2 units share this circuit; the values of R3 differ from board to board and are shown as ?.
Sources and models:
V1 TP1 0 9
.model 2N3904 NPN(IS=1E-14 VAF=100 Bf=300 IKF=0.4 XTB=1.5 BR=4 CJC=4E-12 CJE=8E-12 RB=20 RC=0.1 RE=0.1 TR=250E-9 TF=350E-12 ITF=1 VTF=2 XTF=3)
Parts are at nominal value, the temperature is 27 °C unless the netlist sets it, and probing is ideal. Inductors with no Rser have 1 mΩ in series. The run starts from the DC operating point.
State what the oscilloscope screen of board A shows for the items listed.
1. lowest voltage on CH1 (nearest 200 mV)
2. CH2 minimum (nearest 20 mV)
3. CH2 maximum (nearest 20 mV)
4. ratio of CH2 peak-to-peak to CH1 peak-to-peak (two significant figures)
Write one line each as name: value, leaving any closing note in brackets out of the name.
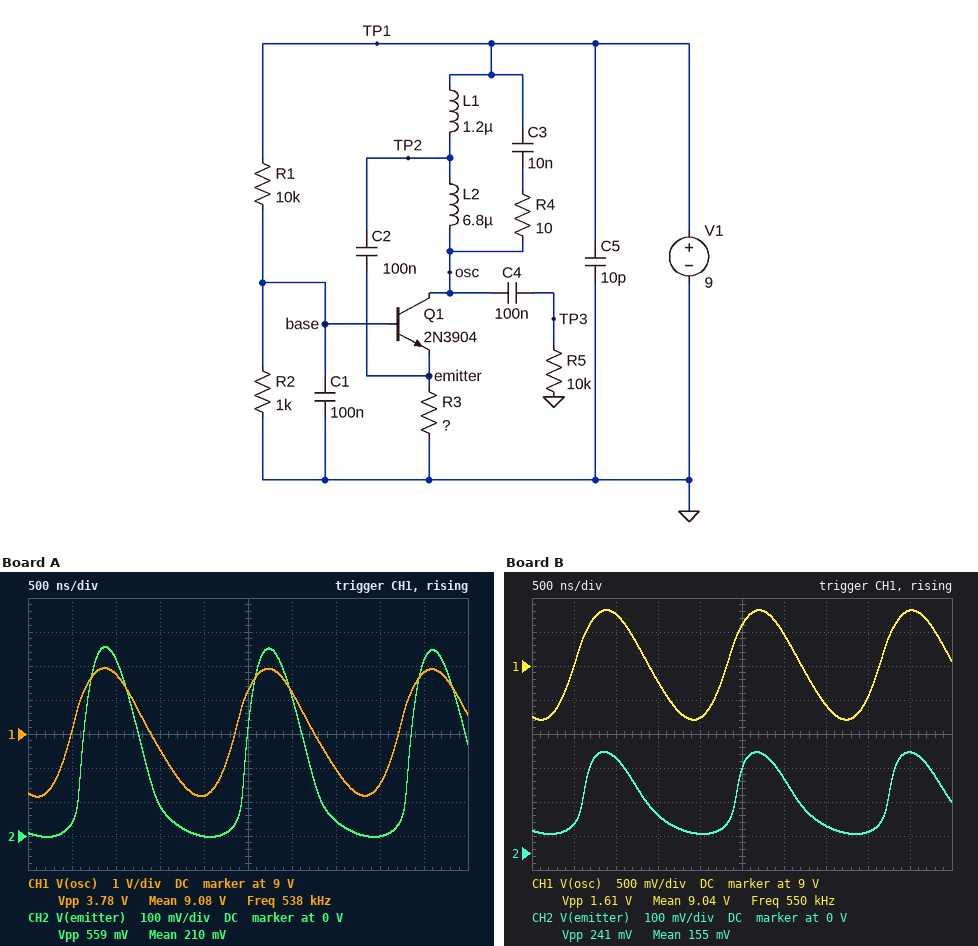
lowest voltage on CH1: 7.2 V
CH2 minimum: 0 V
CH2 maximum: 560 mV
ratio of CH2 peak-to-peak to CH1 peak-to-peak: 0.15
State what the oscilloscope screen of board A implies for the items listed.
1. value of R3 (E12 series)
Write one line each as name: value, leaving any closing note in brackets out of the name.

value of R3: 10 Ω
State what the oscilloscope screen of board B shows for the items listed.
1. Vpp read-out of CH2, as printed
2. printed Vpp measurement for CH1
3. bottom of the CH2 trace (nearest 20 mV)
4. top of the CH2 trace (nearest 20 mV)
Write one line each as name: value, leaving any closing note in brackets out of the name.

Vpp read-out of CH2, as printed: 241 mV
printed Vpp measurement for CH1: 1.61 V
bottom of the CH2 trace: 60 mV
top of the CH2 trace: 300 mV
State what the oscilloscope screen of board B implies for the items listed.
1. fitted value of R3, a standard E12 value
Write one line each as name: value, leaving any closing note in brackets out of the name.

fitted value of R3, a standard E12 value: 18 Ω
